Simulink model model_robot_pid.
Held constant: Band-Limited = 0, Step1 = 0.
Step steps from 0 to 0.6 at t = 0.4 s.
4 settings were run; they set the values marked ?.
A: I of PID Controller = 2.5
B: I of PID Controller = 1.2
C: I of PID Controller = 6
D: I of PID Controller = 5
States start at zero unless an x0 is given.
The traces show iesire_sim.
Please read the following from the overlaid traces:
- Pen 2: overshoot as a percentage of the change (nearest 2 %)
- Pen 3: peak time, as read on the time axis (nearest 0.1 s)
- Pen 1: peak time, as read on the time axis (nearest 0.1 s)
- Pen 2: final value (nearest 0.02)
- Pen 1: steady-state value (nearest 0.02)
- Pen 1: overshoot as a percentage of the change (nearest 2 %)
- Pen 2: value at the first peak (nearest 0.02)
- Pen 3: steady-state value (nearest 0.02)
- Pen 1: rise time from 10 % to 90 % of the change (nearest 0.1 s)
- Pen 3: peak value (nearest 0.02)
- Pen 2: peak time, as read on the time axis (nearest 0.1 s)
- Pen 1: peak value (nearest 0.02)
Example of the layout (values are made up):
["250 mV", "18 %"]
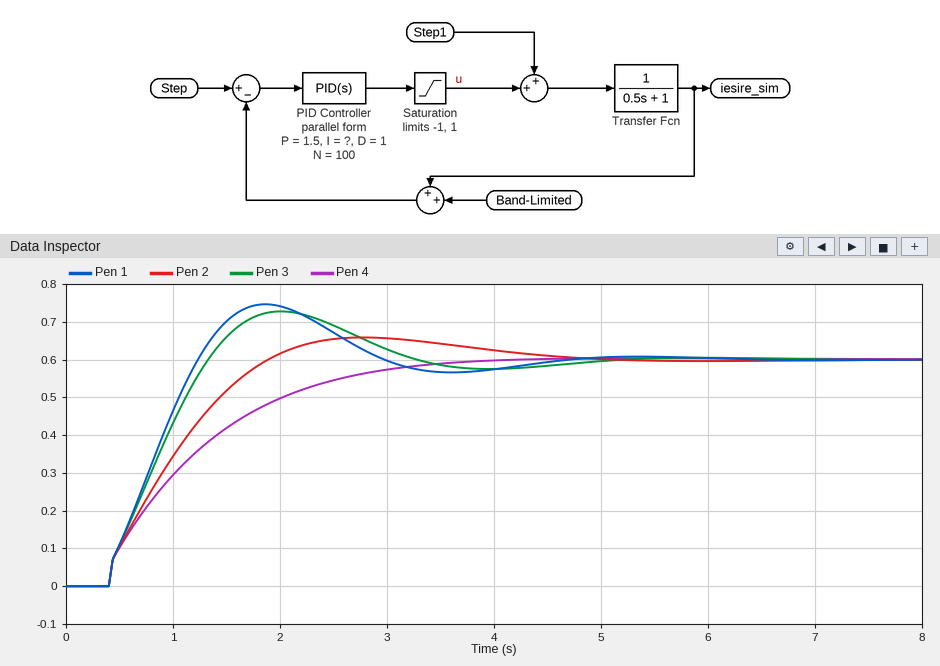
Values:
["10 %", "2.0 s", "1.9 s", "0.60", "0.60", "24 %", "0.66", "0.60", "0.7 s", "0.72", "2.8 s", "0.74"]
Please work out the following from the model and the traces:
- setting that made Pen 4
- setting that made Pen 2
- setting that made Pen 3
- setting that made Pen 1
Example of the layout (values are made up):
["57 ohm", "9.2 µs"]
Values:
["B", "A", "D", "C"]
